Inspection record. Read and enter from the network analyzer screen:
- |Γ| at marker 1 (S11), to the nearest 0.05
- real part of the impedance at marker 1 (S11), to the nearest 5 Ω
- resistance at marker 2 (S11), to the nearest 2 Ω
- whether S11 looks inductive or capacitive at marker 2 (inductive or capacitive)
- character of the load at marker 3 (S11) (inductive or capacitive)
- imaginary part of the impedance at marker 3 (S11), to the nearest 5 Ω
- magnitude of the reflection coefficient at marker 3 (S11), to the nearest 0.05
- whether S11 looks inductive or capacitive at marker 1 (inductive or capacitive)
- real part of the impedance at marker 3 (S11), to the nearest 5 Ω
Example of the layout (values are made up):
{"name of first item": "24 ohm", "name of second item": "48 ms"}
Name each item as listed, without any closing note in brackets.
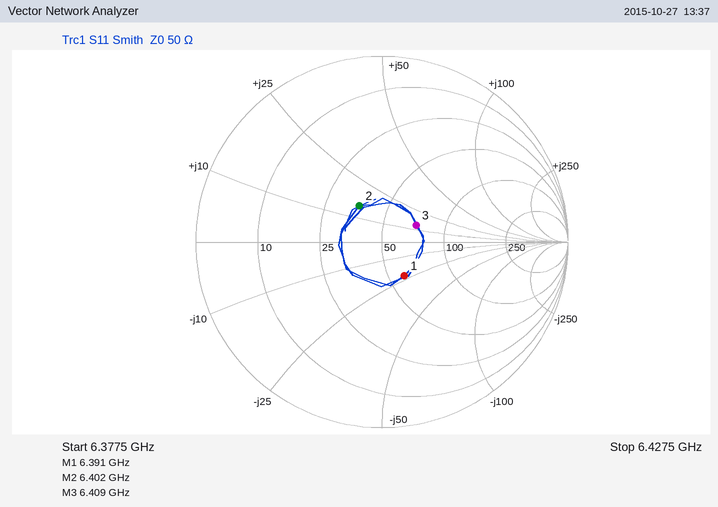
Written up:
{"|Γ| at marker 1 (S11), to the nearest 0.05": "0.20", "real part of the impedance at marker 1 (S11), to the nearest 5 Ω": "60 Ω", "resistance at marker 2 (S11), to the nearest 2 Ω": "36 Ω", "whether S11 looks inductive or capacitive at marker 2": "inductive", "character of the load at marker 3 (S11)": "inductive", "imaginary part of the impedance at marker 3 (S11), to the nearest 5 Ω": "+15 Ω", "magnitude of the reflection coefficient at marker 3 (S11), to the nearest 0.05": "0.20", "whether S11 looks inductive or capacitive at marker 1": "capacitive", "real part of the impedance at marker 3 (S11), to the nearest 5 Ω": "70 Ω"}
